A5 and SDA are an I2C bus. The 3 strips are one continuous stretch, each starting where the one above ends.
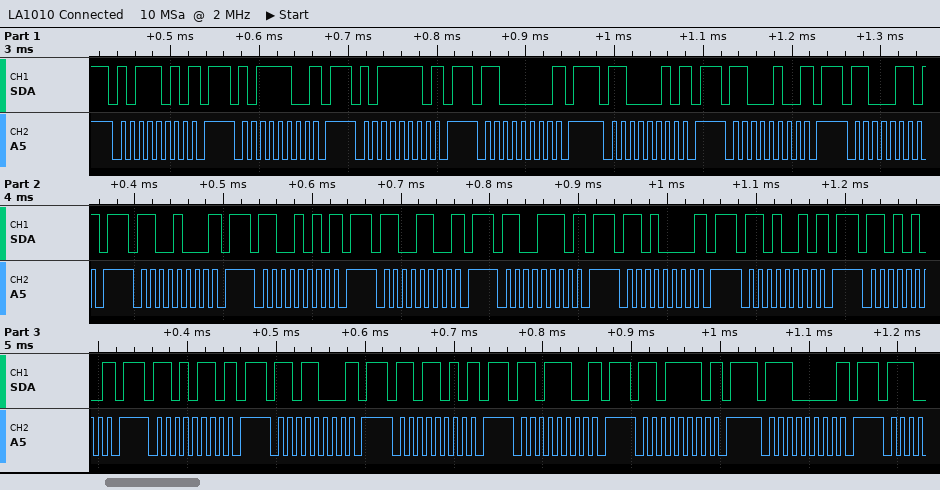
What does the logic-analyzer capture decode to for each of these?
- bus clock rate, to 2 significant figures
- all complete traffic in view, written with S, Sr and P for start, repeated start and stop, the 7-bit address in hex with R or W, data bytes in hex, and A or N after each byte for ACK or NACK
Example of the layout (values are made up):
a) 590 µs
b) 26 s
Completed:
a) 100 kHz
b) S 5DW N P S 5EW N P S 5FW N P S 60W N P S 61W N P S 62W N P S 63W N P S 64W N P S 65W N P S 66W N P S 67W N P S 68W N P S 69W N P S 6AW N P S 6BW N P S 6CW N P S 6DW N P S 6EW N P S 6FW N P S 70W N P
